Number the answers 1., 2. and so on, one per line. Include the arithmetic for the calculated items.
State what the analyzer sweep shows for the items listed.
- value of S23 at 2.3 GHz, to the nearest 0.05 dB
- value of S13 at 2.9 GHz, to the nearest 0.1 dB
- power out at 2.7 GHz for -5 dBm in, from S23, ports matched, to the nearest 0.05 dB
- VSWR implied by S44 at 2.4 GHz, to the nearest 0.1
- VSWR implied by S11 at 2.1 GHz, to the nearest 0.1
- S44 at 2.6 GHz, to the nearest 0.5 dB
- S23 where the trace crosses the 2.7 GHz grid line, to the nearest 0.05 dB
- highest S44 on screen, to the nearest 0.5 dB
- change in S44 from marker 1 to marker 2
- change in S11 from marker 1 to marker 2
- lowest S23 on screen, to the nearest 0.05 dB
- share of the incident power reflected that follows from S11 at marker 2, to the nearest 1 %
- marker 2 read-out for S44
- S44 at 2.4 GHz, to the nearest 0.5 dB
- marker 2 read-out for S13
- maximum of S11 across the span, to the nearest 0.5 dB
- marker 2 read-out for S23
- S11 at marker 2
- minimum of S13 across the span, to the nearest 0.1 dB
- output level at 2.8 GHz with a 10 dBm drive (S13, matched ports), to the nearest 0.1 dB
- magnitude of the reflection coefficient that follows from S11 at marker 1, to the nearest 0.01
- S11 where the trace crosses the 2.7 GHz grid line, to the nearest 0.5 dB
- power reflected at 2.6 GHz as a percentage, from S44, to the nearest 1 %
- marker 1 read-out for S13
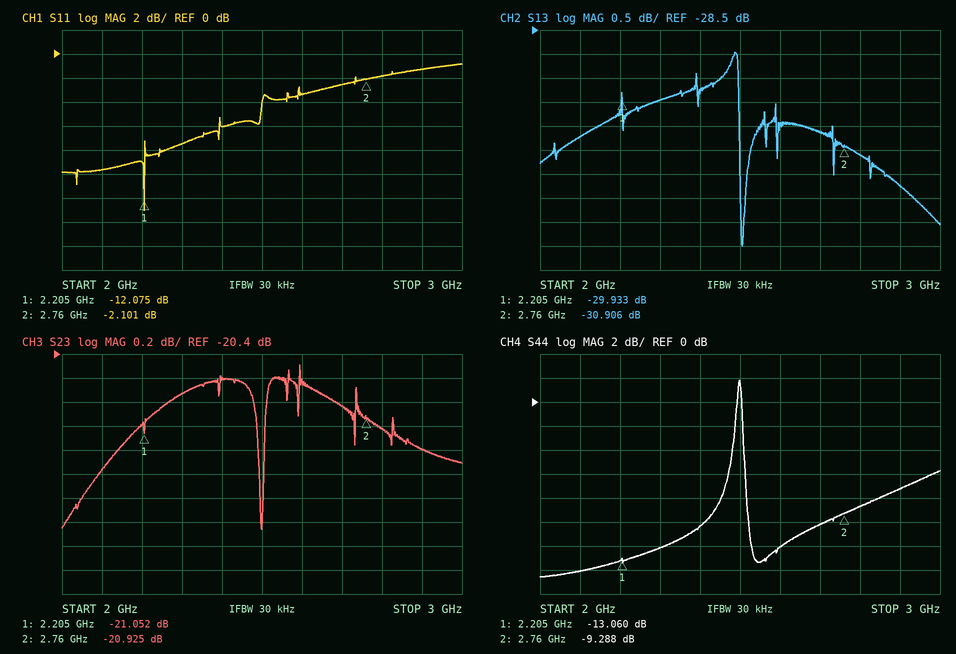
1. -20.75 dB
2. -31.7 dB
3. -5 dBm + (-20.85 dB) = -25.85 dBm
4. |Γ| = 10^(-10.5/20) = 0.2985; VSWR = (1 + 0.2985)/(1 − 0.2985) ≈ 1.9
5. |Γ| = 10^(-9.5/20) = 0.3350; VSWR = (1 + 0.3350)/(1 − 0.3350) ≈ 2.0
6. -12.0 dB
7. -20.85 dB
8. 2.0 dB
9. -9.288 − (-13.06) = 3.772 dB
10. -2.101 − (-12.075) = 9.974 dB
11. -21.85 dB
12. 10^(-2.101/10) ≈ 62 %
13. -9.288 dB
14. -10.5 dB
15. -30.906 dB
16. -1.0 dB
17. -20.925 dB
18. -2.101 dB
19. -33.0 dB
20. 10 dBm + (-31.1 dB) = -21.1 dBm
21. 10^(-12.075/20) ≈ 0.25
22. -2.5 dB
23. 10^(-12/10) ≈ 6 %
24. -29.933 dB
